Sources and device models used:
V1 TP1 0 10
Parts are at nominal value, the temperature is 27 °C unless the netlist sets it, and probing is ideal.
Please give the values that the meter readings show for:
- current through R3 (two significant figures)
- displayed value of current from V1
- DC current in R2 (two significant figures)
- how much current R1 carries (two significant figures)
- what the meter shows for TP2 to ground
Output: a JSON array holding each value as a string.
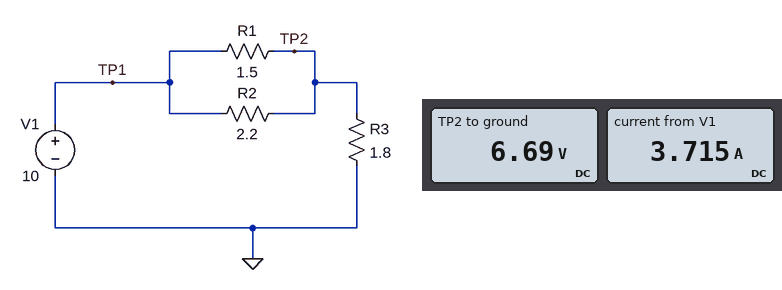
["3.7 A", "3.715 A", "1.5 A", "2.2 A", "6.69 V"]
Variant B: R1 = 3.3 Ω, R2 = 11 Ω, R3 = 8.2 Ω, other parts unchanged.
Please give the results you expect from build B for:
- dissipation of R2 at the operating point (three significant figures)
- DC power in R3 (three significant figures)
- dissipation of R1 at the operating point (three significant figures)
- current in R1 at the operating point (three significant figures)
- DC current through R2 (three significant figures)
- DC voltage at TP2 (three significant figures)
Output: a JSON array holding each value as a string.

["508 mW", "7.11 W", "1.69 W", "716 mA", "215 mA", "7.64 V"]
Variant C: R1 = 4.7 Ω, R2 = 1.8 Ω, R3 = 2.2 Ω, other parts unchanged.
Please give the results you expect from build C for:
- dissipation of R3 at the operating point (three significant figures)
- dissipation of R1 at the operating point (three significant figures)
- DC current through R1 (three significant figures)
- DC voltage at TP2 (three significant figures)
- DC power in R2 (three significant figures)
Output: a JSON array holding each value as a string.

["17.9 W", "2.94 W", "791 mA", "6.28 V", "7.68 W"]
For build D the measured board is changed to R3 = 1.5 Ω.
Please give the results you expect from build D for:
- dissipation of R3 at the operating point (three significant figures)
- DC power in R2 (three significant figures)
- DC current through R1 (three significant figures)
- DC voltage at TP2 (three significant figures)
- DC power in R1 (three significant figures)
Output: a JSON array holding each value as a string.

["26.2 W", "6.32 W", "2.49 A", "6.27 V", "9.27 W"]
